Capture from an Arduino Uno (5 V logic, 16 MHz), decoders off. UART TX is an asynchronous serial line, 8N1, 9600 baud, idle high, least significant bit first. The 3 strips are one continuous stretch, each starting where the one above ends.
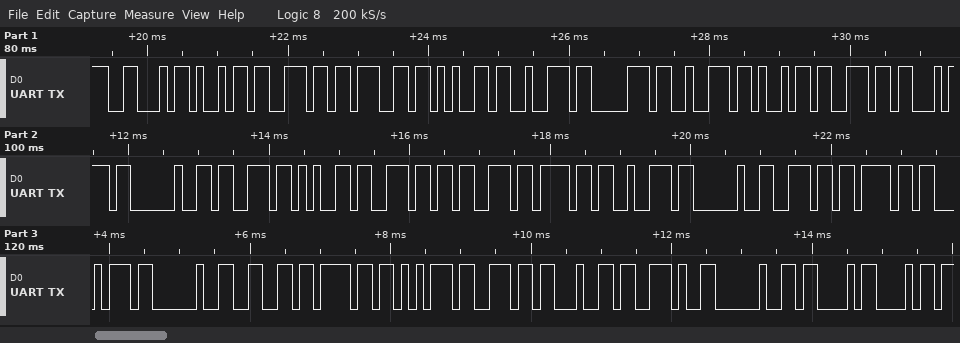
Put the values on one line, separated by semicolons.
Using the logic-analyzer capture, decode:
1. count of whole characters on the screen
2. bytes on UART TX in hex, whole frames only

32; 46 69 6E 67 65 72 70 72 69 6E 74 20 73 65 6E 73 6F 72 20 6E 6F 74 20 66 6F 75 6E 64 2E 20 43 68
